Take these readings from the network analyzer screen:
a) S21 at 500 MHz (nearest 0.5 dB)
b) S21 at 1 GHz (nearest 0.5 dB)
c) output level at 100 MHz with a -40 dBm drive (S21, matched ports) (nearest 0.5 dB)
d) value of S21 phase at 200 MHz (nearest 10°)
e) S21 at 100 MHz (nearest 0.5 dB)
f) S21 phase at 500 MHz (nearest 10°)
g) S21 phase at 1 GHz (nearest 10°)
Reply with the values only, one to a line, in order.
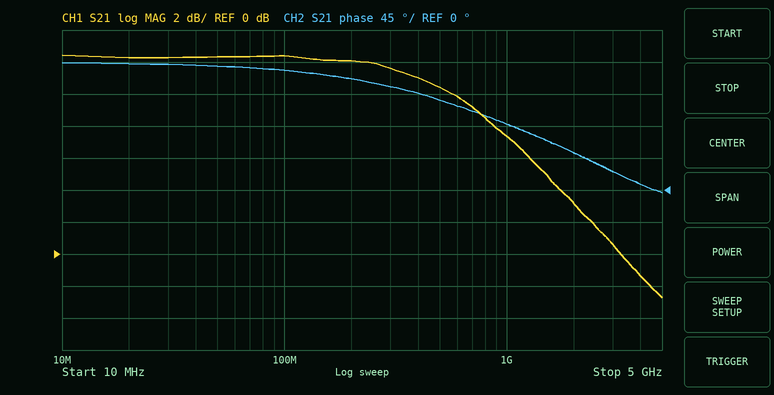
10.5 dB
7.5 dB
-27.5 dBm
160°
12.5 dB
130°
90°
